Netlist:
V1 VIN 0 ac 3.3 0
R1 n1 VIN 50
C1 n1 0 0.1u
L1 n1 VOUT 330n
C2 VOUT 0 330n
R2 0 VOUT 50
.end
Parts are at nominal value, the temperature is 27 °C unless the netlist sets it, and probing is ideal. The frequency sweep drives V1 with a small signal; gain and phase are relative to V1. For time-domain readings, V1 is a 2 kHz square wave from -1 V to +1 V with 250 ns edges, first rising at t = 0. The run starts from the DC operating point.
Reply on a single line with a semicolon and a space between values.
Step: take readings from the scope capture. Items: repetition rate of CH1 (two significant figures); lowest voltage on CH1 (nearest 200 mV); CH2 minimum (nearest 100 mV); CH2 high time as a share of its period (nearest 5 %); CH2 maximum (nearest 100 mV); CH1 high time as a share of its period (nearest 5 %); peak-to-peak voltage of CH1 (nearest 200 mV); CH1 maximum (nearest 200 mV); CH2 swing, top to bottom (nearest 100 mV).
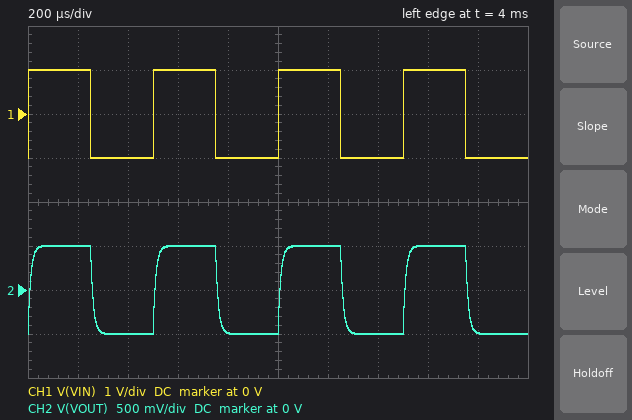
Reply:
2.0 kHz; -1.0 V; -500 mV; 50 %; 500 mV; 50 %; 2.0 V; 1.0 V; 1.0 V
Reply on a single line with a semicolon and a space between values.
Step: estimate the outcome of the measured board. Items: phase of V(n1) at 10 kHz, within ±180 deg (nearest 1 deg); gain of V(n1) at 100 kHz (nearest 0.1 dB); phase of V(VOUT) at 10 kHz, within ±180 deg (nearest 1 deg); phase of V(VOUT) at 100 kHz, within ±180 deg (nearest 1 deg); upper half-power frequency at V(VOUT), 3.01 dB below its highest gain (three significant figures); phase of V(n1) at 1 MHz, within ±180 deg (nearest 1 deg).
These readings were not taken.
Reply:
-34 deg; -23.0 dB; -34 deg; -82 deg; 14.8 kHz; 0 deg
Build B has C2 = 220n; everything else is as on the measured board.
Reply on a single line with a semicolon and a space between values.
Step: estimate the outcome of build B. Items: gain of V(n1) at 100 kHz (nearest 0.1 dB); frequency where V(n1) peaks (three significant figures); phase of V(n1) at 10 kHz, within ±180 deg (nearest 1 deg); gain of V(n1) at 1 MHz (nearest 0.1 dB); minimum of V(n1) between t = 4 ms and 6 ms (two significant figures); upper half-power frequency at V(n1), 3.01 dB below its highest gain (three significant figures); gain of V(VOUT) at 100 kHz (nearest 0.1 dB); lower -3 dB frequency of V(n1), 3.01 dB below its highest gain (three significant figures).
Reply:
-20.4 dB; 1.06 MHz; -27 deg; -15.2 dB; -500 mV; 1.07 MHz; -20.1 dB; 1.04 MHz
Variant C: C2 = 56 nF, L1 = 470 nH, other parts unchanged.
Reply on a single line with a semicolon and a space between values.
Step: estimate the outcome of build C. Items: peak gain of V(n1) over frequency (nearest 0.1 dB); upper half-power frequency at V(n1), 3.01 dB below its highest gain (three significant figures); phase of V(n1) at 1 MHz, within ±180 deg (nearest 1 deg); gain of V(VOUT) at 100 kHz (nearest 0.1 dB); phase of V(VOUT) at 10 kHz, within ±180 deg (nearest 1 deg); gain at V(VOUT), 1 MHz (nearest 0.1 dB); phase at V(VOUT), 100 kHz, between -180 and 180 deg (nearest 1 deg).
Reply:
-6.0 dB; 40.8 kHz; 30 deg; -14.4 dB; -14 deg; -24.3 dB; -68 deg
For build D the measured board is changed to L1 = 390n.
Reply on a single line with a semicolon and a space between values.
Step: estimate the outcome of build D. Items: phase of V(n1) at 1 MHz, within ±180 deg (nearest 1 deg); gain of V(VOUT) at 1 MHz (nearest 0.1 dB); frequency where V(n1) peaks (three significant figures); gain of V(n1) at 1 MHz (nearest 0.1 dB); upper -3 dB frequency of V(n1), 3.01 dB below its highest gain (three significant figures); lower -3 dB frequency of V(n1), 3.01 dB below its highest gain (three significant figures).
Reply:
-80 deg; -27.9 dB; 920 kHz; -15.7 dB; 934 kHz; 907 kHz
